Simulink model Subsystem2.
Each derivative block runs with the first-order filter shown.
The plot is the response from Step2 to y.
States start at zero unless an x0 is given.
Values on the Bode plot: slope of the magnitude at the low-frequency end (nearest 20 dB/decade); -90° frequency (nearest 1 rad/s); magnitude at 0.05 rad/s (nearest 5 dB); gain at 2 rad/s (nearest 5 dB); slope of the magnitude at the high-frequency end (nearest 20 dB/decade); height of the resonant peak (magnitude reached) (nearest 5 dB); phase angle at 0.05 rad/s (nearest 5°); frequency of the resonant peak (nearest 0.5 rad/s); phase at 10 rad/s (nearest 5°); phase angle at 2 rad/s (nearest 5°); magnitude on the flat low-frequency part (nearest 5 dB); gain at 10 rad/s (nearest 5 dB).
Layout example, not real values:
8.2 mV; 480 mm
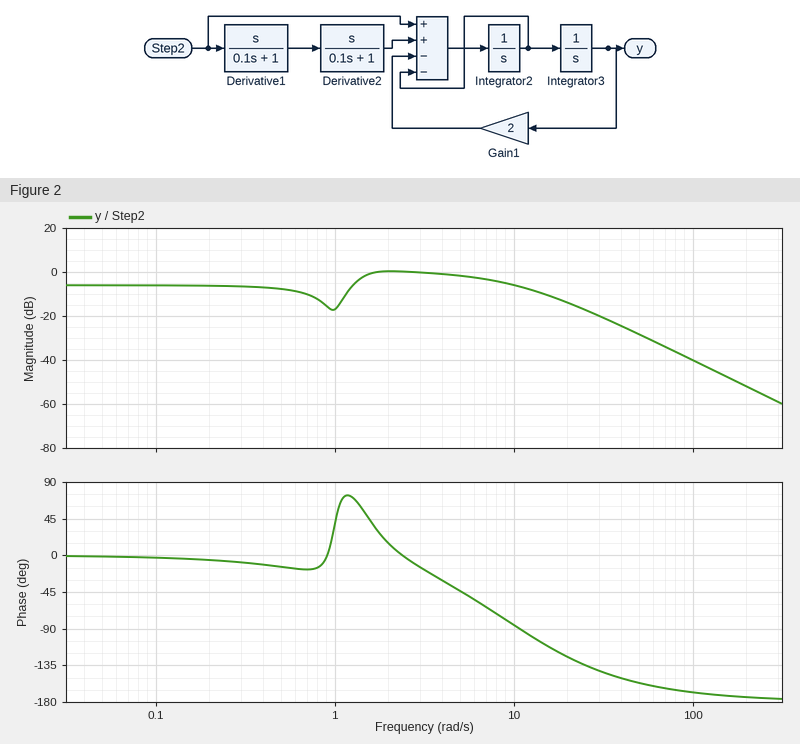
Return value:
0 dB/decade; 11 rad/s; -5 dB; 0 dB; -40 dB/decade; 0 dB; 0°; 2.0 rad/s; -85°; 15°; -5 dB; -5 dB
